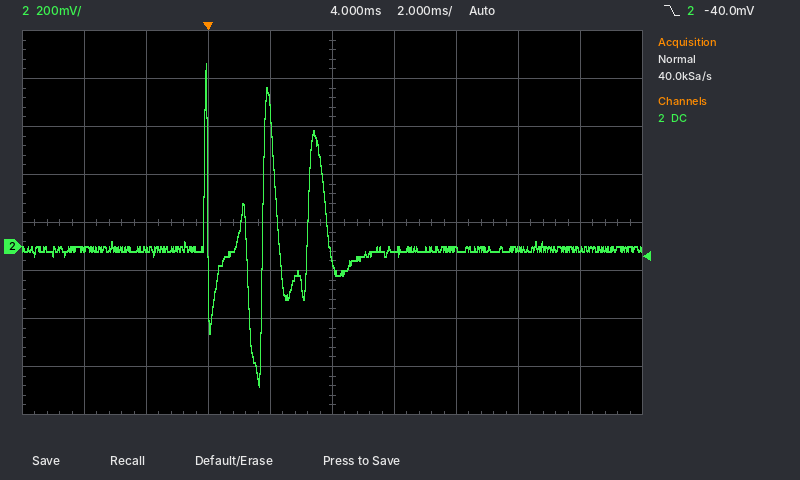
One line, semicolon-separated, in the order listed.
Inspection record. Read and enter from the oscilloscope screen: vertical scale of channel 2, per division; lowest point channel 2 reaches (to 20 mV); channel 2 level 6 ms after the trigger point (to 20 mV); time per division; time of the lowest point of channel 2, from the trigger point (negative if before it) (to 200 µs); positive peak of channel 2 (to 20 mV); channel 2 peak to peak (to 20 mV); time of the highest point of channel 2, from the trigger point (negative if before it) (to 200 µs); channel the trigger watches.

200 mV; -580 mV; -20 mV; 2 ms; +1.6 ms; 760 mV; 1.34 V; 0.0 ms; channel 2
